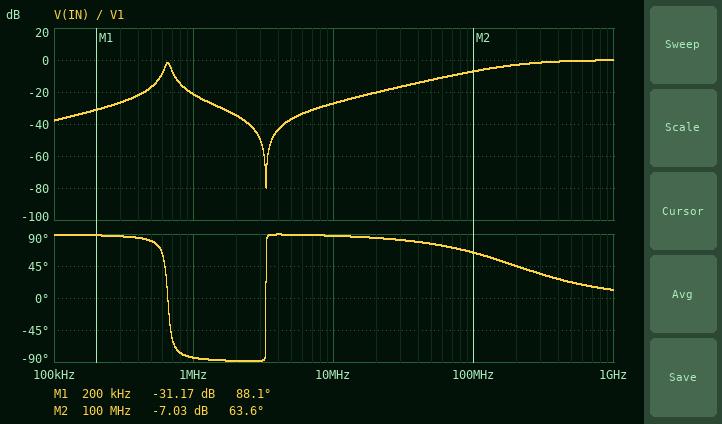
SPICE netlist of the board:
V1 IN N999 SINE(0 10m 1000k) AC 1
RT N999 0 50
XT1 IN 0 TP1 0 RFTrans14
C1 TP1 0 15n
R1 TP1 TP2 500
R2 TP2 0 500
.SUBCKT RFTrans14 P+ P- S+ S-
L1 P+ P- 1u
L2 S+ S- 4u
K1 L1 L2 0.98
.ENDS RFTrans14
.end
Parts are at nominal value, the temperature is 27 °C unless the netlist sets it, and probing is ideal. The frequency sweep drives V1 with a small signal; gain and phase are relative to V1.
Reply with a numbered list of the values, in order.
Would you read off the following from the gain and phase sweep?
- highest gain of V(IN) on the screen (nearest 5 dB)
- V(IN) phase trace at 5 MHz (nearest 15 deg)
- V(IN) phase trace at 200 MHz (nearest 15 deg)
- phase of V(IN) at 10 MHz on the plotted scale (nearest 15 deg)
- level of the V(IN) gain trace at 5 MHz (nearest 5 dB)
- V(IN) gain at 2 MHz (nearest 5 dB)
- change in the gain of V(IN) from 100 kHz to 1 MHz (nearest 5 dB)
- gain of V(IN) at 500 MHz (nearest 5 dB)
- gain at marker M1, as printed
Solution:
1. 0 dB
2. 90 deg
3. 45 deg
4. 90 deg
5. -35 dB
6. -35 dB
7. 15 dB
8. 0 dB
9. -31.17 dB
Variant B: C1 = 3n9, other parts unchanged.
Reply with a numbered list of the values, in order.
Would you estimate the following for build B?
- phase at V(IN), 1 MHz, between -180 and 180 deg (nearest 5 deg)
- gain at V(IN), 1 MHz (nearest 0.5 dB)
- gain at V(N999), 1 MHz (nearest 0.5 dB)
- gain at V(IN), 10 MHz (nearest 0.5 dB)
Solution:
1. 70 deg
2. -10.5 dB
3. -0.5 dB
4. -30.5 dB
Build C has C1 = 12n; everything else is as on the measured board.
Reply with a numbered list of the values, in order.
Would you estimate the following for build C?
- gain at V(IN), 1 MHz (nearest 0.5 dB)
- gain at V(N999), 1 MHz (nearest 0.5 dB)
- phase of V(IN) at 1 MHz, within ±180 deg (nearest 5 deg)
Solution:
1. -18.0 dB
2. 0 dB
3. -80 deg
